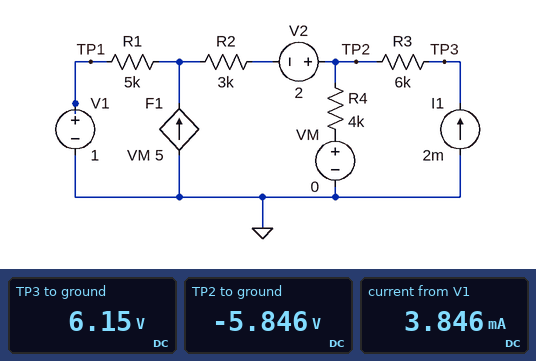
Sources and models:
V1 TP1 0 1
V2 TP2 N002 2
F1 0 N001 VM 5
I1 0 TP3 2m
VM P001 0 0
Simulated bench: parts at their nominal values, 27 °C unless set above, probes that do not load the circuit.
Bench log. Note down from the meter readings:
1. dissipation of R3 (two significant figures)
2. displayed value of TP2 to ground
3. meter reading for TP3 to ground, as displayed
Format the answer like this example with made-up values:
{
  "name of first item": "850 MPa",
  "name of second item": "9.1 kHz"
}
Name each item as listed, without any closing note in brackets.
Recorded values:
{
  "dissipation of R3": "24 mW",
  "displayed value of TP2 to ground": "-5.846 V",
  "meter reading for TP3 to ground, as displayed": "6.15 V"
}
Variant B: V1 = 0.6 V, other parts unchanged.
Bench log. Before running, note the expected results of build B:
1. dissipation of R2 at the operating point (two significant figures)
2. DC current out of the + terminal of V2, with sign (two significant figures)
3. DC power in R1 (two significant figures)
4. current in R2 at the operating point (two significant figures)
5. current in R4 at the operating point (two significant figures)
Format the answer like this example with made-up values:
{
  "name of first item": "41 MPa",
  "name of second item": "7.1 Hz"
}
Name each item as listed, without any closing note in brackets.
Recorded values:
{
  "dissipation of R2 at the operating point": "35 mW",
  "DC current out of the + terminal of V2, with sign": "-3.4 mA",
  "DC power in R1": "69 mW",
  "current in R2 at the operating point": "3.4 mA",
  "current in R4 at the operating point": "1.4 mA"
}
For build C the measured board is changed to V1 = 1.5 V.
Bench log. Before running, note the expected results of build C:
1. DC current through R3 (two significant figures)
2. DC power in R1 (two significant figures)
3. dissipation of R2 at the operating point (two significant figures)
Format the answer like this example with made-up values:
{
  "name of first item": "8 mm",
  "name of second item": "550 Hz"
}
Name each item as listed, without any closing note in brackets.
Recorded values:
{
  "DC current through R3": "2.0 mA",
  "DC power in R1": "80 mW",
  "dissipation of R2 at the operating point": "37 mW"
}
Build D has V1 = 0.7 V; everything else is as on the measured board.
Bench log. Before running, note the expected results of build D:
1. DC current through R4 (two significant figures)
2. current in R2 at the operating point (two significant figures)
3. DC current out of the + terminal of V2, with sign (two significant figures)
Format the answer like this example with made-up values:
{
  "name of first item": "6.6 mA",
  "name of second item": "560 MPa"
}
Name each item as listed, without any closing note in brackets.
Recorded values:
{
  "DC current through R4": "1.4 mA",
  "current in R2 at the operating point": "3.4 mA",
  "DC current out of the + terminal of V2, with sign": "-3.4 mA"
}
